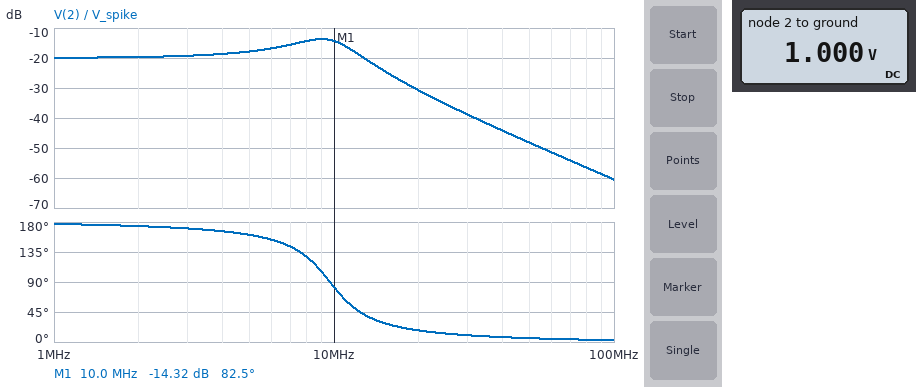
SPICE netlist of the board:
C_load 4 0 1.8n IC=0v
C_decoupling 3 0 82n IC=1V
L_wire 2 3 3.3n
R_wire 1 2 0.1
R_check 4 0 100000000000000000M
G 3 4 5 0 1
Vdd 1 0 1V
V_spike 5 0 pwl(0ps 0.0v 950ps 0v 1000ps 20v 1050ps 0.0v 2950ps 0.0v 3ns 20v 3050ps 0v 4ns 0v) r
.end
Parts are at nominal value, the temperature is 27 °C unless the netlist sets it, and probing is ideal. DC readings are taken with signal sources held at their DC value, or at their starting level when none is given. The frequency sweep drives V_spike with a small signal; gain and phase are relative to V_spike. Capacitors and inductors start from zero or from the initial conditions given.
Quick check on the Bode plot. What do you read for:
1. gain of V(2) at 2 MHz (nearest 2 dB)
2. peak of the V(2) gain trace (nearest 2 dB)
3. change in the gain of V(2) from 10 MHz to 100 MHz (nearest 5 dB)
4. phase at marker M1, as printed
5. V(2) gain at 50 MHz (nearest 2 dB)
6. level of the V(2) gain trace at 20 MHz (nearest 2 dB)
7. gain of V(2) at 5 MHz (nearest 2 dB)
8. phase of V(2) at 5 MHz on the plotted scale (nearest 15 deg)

-20 dB
-14 dB
-45 dB
82.5 deg
-48 dB
-30 dB
-18 dB
165 deg
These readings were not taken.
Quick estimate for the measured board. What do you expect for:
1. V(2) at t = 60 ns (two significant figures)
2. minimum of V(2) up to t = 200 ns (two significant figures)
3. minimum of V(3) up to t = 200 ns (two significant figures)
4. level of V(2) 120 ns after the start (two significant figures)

930 mV
930 mV
880 mV
960 mV
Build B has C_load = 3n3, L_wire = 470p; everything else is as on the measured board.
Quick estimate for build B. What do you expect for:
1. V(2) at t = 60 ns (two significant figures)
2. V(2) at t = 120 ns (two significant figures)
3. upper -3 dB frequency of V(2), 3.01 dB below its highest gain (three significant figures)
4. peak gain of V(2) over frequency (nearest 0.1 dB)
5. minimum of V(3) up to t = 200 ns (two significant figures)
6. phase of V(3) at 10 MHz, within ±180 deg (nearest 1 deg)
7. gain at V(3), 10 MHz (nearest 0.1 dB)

950 mV
950 mV
27.1 MHz
-19.9 dB
940 mV
165 deg
-19.6 dB
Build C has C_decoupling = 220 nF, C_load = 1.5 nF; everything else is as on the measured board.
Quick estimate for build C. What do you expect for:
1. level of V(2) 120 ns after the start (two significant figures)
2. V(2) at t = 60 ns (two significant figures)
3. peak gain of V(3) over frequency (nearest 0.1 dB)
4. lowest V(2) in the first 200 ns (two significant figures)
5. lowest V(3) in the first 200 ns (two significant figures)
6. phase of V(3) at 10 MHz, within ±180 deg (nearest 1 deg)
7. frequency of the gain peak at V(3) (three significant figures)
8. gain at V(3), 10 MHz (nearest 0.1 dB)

940 mV
950 mV
-14.1 dB
940 mV
920 mV
101 deg
5.48 MHz
-20.1 dB
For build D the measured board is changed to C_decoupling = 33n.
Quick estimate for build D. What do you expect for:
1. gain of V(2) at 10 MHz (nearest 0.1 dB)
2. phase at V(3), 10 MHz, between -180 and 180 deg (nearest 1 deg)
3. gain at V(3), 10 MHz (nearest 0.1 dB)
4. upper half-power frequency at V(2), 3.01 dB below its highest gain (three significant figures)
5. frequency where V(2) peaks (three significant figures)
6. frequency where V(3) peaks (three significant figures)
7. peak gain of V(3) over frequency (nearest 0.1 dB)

-15.7 dB
-136 deg
-8.4 dB
17.1 MHz
14.9 MHz
15.2 MHz
0.4 dB
